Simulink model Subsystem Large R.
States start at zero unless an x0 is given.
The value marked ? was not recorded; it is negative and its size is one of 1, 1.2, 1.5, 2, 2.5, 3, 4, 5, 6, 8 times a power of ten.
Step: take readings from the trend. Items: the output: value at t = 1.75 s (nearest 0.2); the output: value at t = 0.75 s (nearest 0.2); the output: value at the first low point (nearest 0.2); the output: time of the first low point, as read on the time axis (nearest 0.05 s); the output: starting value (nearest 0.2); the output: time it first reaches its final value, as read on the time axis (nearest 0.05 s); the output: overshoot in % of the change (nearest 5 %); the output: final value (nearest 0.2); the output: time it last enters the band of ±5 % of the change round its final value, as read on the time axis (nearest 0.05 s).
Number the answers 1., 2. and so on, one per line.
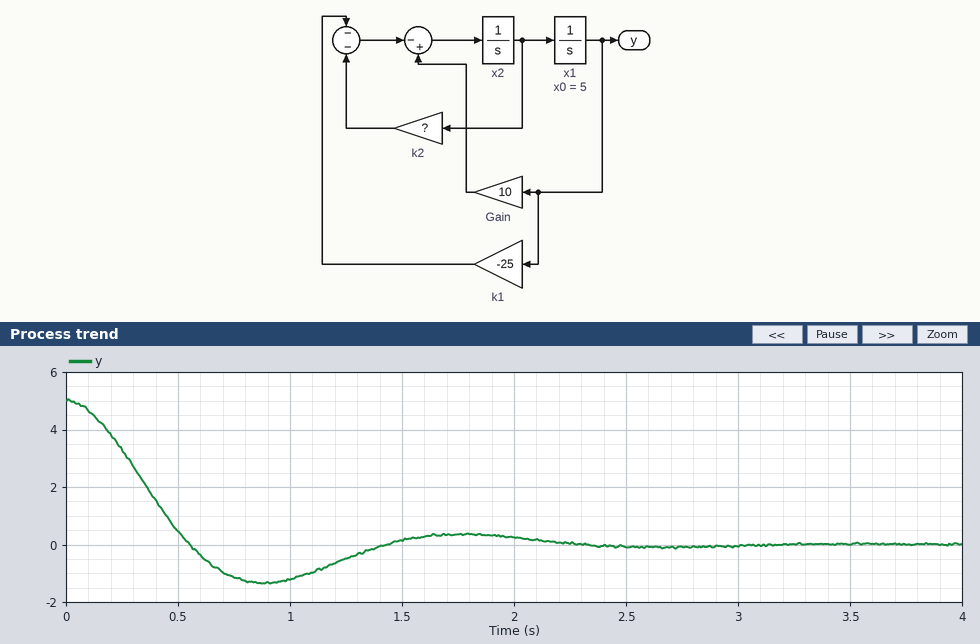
1. 0.4
2. -1.2
3. -1.4
4. 0.90 s
5. 5.0
6. 0.55 s
7. 25 %
8. 0.0
9. 2.00 s
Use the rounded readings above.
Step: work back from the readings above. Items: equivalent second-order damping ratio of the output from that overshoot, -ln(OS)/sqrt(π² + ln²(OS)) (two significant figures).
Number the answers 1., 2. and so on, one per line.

1. 0.40
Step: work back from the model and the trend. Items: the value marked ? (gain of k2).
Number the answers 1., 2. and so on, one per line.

1. -3
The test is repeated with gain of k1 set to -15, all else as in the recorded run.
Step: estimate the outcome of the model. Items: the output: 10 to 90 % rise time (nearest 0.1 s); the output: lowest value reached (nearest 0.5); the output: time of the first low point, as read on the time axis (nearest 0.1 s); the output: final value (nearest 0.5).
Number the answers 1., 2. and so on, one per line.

1. 0.9 s
2. -0.5
3. 1.9 s
4. 0.0
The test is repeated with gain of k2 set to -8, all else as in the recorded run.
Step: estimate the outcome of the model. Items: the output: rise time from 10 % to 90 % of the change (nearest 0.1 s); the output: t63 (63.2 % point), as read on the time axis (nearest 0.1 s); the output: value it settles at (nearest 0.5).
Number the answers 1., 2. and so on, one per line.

1. 0.9 s
2. 0.6 s
3. 0.0
